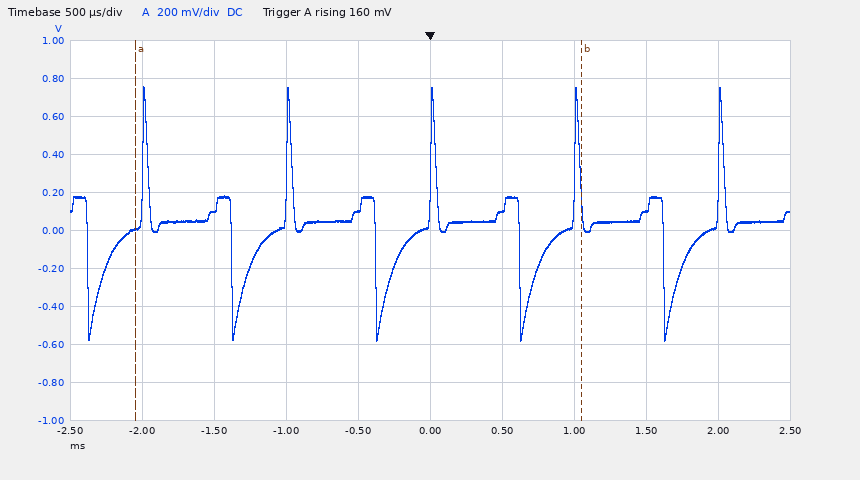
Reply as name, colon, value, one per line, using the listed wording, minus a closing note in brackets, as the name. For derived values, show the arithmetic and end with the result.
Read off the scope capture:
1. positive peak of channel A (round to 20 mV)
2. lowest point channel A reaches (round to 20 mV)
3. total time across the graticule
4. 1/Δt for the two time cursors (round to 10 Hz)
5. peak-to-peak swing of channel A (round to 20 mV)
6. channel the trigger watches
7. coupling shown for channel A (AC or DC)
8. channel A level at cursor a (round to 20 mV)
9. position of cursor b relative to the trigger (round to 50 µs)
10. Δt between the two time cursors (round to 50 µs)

positive peak of channel A: 760 mV
lowest point channel A reaches: -580 mV
total time across the graticule: 5 ms
1/Δt for the two time cursors: 1 / 3.10 ms ≈ 320 Hz
peak-to-peak swing of channel A: 760 mV − (-580 mV) = 1.34 V
channel the trigger watches: channel A
coupling shown for channel A: DC
channel A level at cursor a: 0 mV
position of cursor b relative to the trigger: +1.05 ms
Δt between the two time cursors: 3.10 ms
